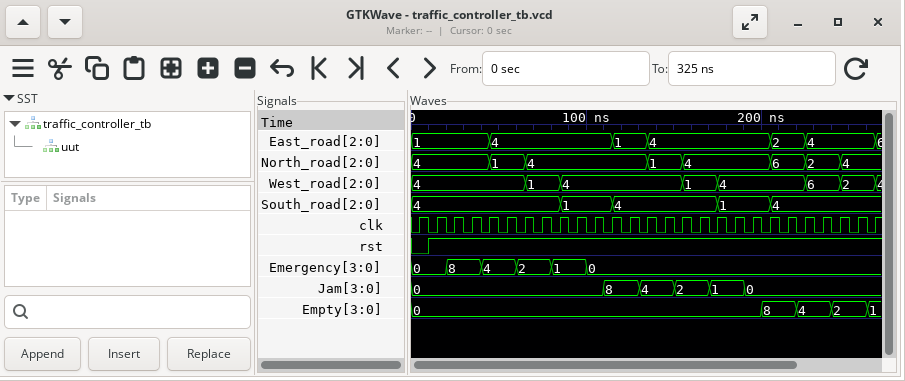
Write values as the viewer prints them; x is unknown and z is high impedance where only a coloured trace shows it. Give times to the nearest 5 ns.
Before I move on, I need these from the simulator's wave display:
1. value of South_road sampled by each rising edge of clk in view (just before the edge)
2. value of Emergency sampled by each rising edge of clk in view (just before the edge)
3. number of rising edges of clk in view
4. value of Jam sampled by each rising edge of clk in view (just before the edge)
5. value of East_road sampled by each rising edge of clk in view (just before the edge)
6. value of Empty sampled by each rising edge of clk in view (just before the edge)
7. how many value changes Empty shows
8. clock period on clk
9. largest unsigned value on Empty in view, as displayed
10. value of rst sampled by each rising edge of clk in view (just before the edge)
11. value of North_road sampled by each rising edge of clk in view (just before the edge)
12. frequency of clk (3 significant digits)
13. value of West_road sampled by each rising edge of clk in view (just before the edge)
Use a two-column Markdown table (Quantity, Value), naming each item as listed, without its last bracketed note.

| Quantity | Value |
|---|---|
| value of South_road sampled by each rising edge of clk in view | 4, 4, 4, 4, 4, 4, 4, 4, 4, 1, 1, 1, 4, 4, 4, 4, 4, 4, 1, 1, 1, 4, 4, 4, 4, 4, 4 |
| value of Emergency sampled by each rising edge of clk in view | 0, 0, 8, 8, 4, 4, 2, 2, 1, 1, 0, 0, 0, 0, 0, 0, 0, 0, 0, 0, 0, 0, 0, 0, 0, 0, 0 |
| number of rising edges of clk in view | 27 |
| value of Jam sampled by each rising edge of clk in view | 0, 0, 0, 0, 0, 0, 0, 0, 0, 0, 0, 8, 8, 4, 4, 2, 2, 1, 1, 0, 0, 0, 0, 0, 0, 0, 0 |
| value of East_road sampled by each rising edge of clk in view | 1, 1, 1, 1, 1, 4, 4, 4, 4, 4, 4, 4, 1, 1, 4, 4, 4, 4, 4, 4, 4, 2, 2, 4, 4, 4, 4 |
| value of Empty sampled by each rising edge of clk in view | 0, 0, 0, 0, 0, 0, 0, 0, 0, 0, 0, 0, 0, 0, 0, 0, 0, 0, 0, 0, 8, 8, 4, 4, 2, 2, 1 |
| how many value changes Empty shows | 4 |
| clock period on clk | 10 ns |
| largest unsigned value on Empty in view, as displayed | 8 |
| value of rst sampled by each rising edge of clk in view | 0 1 1 1 1 1 1 1 1 1 1 1 1 1 1 1 1 1 1 1 1 1 1 1 1 1 1 |
| value of North_road sampled by each rising edge of clk in view | 4, 4, 4, 4, 4, 1, 1, 4, 4, 4, 4, 4, 4, 4, 1, 1, 4, 4, 4, 4, 4, 6, 6, 2, 2, 4, 4 |
| frequency of clk | 100 MHz |
| value of West_road sampled by each rising edge of clk in view | 4, 4, 4, 4, 4, 4, 4, 1, 1, 4, 4, 4, 4, 4, 4, 4, 1, 1, 4, 4, 4, 4, 4, 6, 6, 2, 2 |
